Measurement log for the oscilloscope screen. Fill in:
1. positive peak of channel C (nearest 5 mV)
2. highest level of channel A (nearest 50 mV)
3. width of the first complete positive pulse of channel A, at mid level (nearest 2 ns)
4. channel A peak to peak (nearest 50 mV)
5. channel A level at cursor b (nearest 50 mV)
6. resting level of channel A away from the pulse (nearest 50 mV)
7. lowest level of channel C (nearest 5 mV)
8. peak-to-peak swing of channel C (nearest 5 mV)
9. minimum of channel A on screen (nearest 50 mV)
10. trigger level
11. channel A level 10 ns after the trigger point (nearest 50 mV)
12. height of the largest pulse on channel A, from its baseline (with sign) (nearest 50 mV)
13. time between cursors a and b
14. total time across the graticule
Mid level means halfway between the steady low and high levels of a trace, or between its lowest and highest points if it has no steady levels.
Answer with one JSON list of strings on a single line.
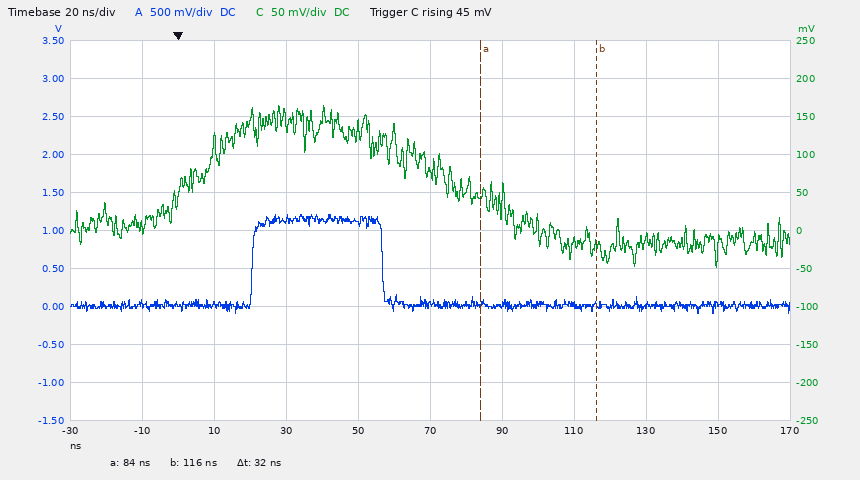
["165 mV", "1.20 V", "36 ns", "1.30 V", "0 mV", "0 mV", "-50 mV", "215 mV", "-100 mV", "45 mV", "0 mV", "+1.20 V", "32 ns", "200 ns"]
